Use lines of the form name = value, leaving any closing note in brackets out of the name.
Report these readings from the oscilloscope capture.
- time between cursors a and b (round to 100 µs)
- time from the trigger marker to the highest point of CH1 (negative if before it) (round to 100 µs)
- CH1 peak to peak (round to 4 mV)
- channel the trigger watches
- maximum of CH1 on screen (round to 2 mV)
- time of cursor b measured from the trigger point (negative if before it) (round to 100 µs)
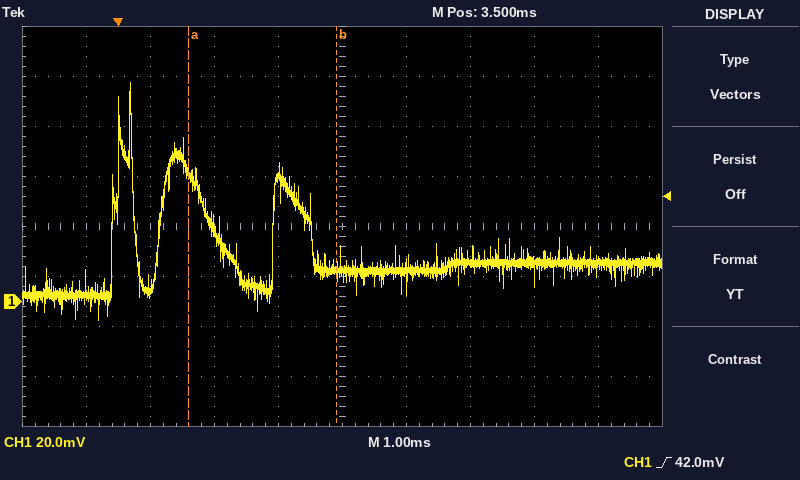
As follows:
time between cursors a and b = 2.3 ms
time from the trigger marker to the highest point of CH1 (negative if before it) = +200 µs
CH1 peak to peak = 96 mV
channel the trigger watches = CH1
maximum of CH1 on screen = 88 mV
time of cursor b measured from the trigger point (negative if before it) = +3.4 ms
